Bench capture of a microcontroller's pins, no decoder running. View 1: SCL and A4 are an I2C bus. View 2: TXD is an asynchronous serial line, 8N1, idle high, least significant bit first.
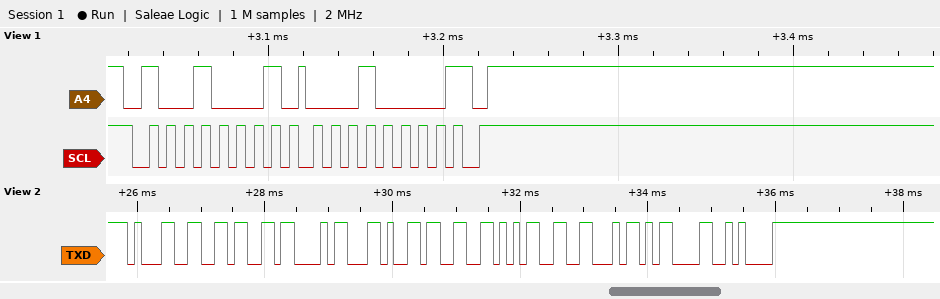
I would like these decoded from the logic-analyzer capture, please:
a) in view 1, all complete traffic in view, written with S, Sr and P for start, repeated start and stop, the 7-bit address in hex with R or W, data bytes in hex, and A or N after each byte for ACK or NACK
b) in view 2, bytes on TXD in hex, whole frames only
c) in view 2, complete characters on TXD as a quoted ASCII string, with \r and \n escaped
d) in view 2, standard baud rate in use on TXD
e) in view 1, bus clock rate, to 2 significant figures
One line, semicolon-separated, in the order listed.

S 48R A 10 N P; 31 36 43 2C 33 35 46 0D 0A; "16C,35F\r\n"; 9600 baud; 100 kHz
